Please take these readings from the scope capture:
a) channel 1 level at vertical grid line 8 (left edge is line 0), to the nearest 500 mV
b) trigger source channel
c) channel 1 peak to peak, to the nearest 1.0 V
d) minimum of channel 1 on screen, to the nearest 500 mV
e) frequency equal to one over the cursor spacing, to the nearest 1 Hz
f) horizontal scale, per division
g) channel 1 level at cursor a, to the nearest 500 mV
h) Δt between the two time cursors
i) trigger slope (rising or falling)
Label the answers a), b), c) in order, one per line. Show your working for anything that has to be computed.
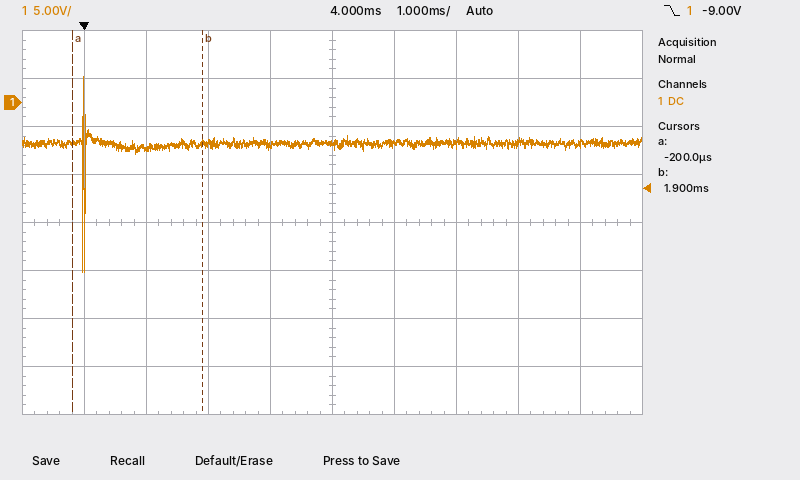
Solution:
a) -4.0 V
b) channel 1
c) 20.0 V
d) -17.5 V
e) 1 / 2.1 ms ≈ 476 Hz
f) 1 ms
g) -4.0 V
h) 1.9 ms − (-200 µs) = 2.1 ms
i) falling
